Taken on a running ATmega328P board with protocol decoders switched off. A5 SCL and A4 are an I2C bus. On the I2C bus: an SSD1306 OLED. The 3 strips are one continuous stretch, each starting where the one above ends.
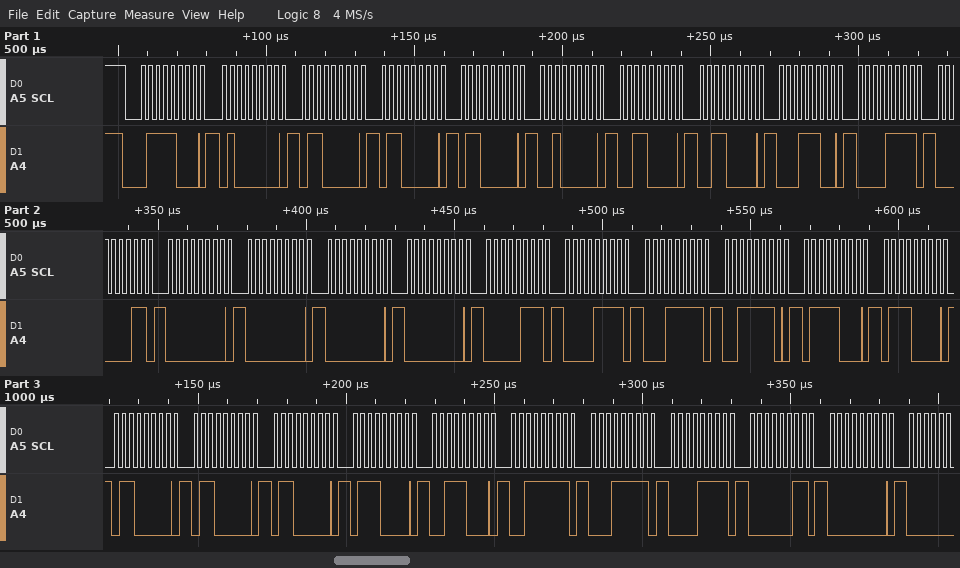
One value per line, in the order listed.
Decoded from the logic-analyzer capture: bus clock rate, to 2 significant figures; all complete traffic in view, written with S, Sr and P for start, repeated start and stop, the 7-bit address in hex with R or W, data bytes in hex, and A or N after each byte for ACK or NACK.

400 kHz
S 3CW A 40 A 60 A 60 A 60 A 20 A 30 A 30 A 1C A 0F A 03 A 00 A 00 A 00 A 00 A 07 A 0F A 1F A 3E A 78 A 70 A 60 A 60 A 60 A 70 A 38 A 3F A 1F A 0F A 03 A 00 A
